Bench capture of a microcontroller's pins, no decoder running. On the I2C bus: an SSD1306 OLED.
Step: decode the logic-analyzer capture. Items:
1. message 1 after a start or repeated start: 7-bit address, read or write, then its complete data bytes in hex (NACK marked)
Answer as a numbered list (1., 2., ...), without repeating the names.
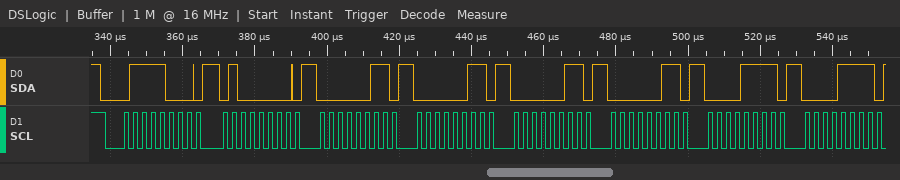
1. 0x3C write: 40 03 03 03 03 0F 0F
